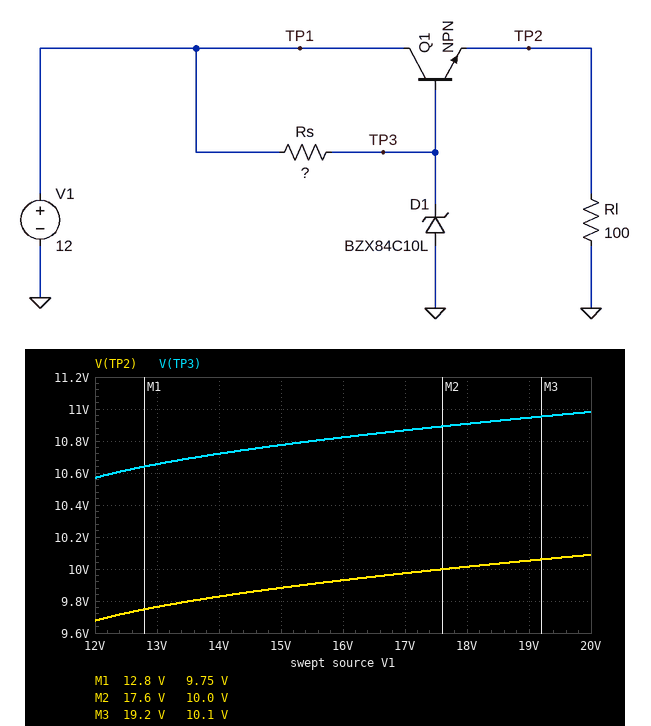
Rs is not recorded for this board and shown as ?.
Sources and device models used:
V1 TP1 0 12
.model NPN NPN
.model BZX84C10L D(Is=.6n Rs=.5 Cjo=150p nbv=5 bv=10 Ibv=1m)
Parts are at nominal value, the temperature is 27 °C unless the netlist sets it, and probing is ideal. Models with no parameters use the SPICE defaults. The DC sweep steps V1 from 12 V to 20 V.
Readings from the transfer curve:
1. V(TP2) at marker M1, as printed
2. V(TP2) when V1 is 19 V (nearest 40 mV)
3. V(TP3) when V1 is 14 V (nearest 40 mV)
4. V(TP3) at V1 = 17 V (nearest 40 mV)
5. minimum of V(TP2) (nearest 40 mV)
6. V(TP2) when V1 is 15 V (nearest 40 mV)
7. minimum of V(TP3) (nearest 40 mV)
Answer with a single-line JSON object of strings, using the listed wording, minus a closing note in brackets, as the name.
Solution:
{"V(TP2) at marker M1, as printed": "9.75 V", "V(TP2) when V1 is 19 V": "10.04 V", "V(TP3) when V1 is 14 V": "10.72 V", "V(TP3) at V1 = 17 V": "10.88 V", "minimum of V(TP2)": "9.68 V", "V(TP2) when V1 is 15 V": "9.88 V", "minimum of V(TP3)": "10.56 V"}
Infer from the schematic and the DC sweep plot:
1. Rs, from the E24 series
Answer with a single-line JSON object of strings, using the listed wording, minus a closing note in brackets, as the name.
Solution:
{"Rs, from the E24 series": "22 Ω"}
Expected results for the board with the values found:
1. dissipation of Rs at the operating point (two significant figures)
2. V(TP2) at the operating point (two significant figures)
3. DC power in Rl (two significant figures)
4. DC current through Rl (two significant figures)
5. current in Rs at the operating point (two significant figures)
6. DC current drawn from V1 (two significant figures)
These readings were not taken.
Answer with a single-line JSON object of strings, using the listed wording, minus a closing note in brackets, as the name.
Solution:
{"dissipation of Rs at the operating point": "93 mW", "V(TP2) at the operating point": "9.7 V", "DC power in Rl": "940 mW", "DC current through Rl": "97 mA", "current in Rs at the operating point": "65 mA", "DC current drawn from V1": "160 mA"}
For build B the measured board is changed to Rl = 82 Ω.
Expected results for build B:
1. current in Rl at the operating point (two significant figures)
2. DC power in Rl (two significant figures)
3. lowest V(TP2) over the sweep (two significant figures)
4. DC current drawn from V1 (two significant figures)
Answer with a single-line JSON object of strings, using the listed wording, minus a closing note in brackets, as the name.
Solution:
{"current in Rl at the operating point": "120 mA", "DC power in Rl": "1.1 W", "lowest V(TP2) over the sweep": "9.7 V", "DC current drawn from V1": "180 mA"}
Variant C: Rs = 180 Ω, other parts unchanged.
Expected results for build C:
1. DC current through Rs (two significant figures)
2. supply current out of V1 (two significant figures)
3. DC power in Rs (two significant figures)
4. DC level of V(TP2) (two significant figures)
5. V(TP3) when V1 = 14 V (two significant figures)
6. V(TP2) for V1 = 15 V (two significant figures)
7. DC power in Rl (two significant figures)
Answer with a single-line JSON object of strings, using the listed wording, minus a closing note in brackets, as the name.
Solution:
{"DC current through Rs": "9.5 mA", "supply current out of V1": "100 mA", "DC power in Rs": "16 mW", "DC level of V(TP2)": "9.4 V", "V(TP3) when V1 = 14 V": "10 V", "V(TP2) for V1 = 15 V": "9.5 V", "DC power in Rl": "880 mW"}
